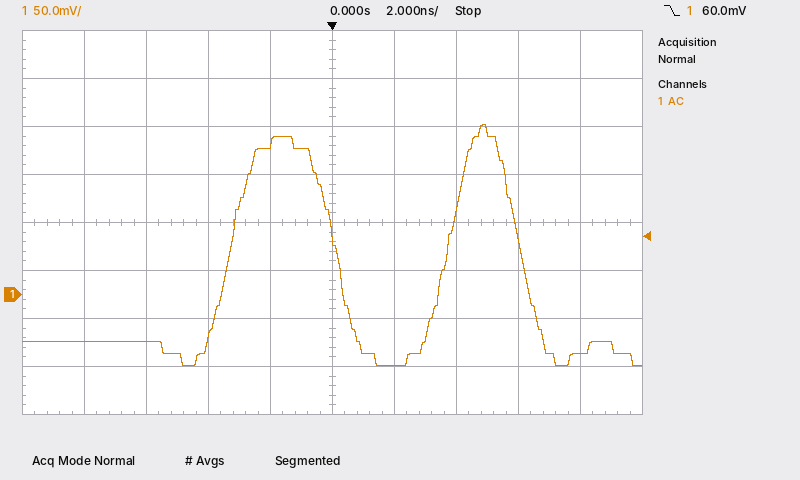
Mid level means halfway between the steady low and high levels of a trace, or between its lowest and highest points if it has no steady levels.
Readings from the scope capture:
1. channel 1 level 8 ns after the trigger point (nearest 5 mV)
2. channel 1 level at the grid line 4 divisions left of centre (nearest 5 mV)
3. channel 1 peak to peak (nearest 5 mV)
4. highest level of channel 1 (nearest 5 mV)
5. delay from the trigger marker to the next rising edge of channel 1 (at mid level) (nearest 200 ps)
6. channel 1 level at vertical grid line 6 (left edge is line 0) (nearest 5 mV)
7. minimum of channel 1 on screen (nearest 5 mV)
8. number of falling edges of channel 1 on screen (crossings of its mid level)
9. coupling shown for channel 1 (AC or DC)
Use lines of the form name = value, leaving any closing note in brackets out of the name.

channel 1 level 8 ns after the trigger point = -60 mV
channel 1 level at the grid line 4 divisions left of centre = -50 mV
channel 1 peak to peak = 250 mV
highest level of channel 1 = 175 mV
delay from the trigger marker to the next rising edge of channel 1 (at mid level) = 3.8 ns
channel 1 level at vertical grid line 6 (left edge is line 0) = -75 mV
minimum of channel 1 on screen = -75 mV
number of falling edges of channel 1 on screen = 2
coupling shown for channel 1 = AC
